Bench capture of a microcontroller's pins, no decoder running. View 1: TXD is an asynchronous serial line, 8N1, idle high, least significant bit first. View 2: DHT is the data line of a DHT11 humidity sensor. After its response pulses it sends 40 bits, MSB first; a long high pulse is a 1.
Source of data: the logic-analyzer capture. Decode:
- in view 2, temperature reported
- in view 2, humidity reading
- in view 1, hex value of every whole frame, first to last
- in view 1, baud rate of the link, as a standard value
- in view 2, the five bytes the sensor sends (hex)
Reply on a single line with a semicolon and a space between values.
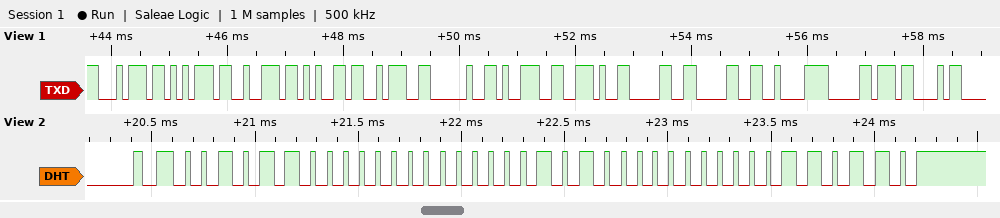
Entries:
10.0 °C; 44 %; 74 75 72 65 3A 20 39 2E 30 30 C2 B0 43; 9600 baud; 2C 00 0A 00 36
